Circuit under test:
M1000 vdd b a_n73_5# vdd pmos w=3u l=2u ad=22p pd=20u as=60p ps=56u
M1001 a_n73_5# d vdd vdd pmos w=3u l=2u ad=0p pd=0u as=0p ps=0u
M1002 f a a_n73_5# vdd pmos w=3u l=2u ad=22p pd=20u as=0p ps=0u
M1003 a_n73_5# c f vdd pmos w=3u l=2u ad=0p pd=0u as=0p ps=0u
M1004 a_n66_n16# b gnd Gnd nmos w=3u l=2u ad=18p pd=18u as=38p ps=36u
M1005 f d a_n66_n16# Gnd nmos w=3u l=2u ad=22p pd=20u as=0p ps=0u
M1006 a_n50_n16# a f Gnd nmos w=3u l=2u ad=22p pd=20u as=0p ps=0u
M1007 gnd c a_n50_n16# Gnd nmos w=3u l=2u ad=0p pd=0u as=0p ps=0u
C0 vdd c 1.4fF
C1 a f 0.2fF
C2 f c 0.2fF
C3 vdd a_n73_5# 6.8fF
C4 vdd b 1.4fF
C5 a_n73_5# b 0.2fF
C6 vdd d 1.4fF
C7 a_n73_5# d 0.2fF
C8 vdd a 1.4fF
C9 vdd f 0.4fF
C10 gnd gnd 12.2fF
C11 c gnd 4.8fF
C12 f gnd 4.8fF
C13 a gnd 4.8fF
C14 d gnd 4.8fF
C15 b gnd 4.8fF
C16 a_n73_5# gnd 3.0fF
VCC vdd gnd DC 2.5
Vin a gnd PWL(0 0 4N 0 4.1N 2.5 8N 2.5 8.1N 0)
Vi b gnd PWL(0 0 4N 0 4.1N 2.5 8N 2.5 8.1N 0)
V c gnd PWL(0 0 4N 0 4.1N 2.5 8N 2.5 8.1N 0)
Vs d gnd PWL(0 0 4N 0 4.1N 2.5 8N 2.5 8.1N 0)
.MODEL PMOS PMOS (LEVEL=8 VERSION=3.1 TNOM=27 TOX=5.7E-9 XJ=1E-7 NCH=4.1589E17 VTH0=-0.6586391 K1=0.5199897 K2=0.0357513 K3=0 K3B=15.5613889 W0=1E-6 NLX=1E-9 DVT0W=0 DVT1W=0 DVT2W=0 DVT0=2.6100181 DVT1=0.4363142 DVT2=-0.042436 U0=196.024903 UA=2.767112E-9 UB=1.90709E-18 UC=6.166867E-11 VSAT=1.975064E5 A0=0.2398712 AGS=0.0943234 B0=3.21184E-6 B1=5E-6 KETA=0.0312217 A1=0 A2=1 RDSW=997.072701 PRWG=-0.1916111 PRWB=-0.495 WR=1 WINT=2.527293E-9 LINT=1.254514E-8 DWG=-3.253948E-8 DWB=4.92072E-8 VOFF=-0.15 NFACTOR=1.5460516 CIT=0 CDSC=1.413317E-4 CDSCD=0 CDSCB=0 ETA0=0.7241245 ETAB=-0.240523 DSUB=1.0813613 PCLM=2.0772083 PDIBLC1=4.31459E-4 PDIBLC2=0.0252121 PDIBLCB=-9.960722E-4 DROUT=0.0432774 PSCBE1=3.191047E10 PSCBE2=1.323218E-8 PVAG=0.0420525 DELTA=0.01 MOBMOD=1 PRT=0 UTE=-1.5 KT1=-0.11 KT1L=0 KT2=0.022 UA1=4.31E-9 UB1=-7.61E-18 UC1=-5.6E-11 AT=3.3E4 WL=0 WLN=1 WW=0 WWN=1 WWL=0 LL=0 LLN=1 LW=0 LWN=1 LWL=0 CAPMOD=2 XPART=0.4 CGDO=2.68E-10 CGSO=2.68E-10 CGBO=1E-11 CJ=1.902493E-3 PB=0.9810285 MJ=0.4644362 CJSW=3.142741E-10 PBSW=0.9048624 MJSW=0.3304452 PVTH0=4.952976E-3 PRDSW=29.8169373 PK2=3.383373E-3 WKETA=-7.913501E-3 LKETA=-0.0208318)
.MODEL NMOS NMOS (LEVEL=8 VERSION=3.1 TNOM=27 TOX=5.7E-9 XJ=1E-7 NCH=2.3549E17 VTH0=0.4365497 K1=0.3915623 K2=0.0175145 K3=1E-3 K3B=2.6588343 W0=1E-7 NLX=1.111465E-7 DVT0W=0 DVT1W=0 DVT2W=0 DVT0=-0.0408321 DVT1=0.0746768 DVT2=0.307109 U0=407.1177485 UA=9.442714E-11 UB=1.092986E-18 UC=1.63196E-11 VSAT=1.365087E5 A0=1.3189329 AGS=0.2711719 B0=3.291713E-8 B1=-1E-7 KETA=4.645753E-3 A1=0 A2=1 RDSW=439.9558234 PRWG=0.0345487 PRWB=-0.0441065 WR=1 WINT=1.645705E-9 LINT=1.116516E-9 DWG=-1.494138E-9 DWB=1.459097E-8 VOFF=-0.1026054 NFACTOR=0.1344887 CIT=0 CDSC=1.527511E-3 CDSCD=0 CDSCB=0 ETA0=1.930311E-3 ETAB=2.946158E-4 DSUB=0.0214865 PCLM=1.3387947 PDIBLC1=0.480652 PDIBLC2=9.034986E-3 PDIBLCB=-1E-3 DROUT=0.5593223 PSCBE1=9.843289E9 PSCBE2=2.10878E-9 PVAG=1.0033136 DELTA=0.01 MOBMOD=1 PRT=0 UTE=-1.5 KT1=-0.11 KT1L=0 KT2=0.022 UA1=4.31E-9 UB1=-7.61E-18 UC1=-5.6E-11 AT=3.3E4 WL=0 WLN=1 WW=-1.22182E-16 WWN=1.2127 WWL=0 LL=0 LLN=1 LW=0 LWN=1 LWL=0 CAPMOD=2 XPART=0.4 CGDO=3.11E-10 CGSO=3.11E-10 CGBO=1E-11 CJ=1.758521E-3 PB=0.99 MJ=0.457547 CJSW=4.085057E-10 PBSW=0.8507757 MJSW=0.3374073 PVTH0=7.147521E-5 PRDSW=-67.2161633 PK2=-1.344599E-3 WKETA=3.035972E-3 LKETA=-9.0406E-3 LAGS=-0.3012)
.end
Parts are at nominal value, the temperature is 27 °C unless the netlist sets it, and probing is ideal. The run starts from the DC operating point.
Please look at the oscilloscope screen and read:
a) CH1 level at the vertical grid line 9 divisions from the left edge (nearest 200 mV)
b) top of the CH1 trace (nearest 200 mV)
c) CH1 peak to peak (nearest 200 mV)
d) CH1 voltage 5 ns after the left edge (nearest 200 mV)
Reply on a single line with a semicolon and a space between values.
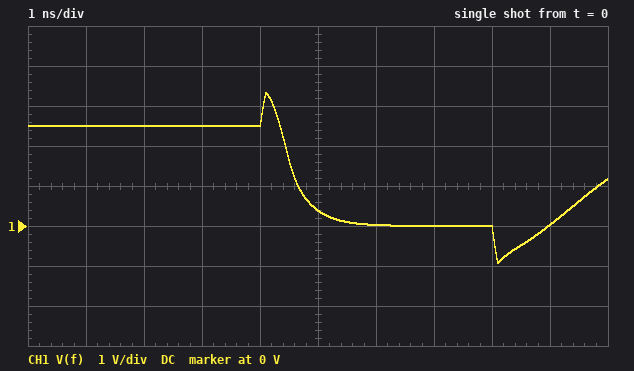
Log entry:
0 V; 3.4 V; 4.2 V; 400 mV
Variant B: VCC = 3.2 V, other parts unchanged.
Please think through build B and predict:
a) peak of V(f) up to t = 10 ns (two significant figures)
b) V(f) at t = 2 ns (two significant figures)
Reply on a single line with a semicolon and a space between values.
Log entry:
4.0 V; 3.2 V
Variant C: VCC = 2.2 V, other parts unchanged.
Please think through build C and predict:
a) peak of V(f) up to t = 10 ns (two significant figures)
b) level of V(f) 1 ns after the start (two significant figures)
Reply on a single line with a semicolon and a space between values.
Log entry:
3.0 V; 2.2 V
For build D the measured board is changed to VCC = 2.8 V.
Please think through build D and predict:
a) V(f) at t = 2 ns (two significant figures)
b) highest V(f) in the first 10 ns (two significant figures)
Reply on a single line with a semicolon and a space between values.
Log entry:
2.8 V; 3.6 V
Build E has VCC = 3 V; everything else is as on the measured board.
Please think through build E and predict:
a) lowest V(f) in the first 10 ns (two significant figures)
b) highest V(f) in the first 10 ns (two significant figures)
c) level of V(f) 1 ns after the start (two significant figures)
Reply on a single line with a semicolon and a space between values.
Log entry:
-910 mV; 3.8 V; 3.0 V
